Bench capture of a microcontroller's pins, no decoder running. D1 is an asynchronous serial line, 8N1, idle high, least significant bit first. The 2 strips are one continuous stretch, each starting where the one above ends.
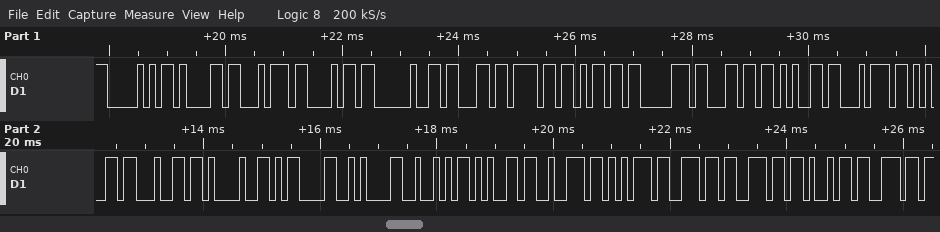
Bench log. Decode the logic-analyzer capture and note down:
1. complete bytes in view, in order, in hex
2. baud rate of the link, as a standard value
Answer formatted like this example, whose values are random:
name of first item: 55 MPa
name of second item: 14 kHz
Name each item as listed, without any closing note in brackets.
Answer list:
complete bytes in view, in order, in hex: 50 61 74 68 20 63 6F 6D 70 6C 65 74 65 64 21 0D 0A 52 65 72 75 6E 6E 69 6E
baud rate of the link, as a standard value: 9600 baud
